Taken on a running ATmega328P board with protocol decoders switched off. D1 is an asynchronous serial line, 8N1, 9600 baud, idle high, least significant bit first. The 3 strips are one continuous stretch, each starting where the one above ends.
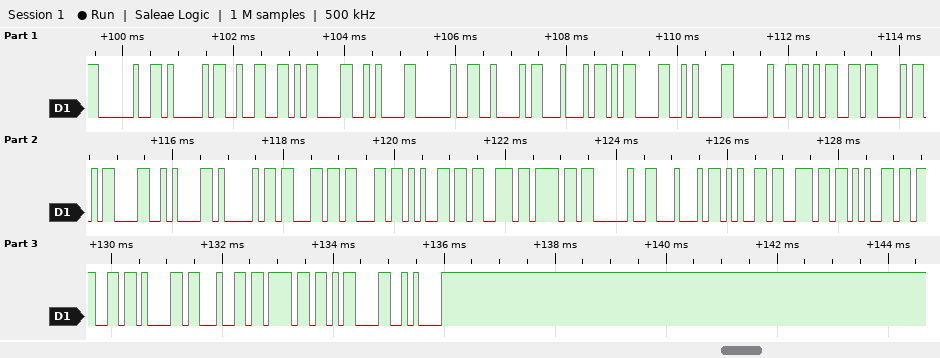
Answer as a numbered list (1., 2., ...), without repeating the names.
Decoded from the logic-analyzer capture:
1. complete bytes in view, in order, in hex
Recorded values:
1. 20 41 32 0D 0A 20 42 44 0D 0A 20 35 43 0D 0A 41 63 63 65 73 6F 20 44 65 6E 65 67 61 64 6F 0D 0A
